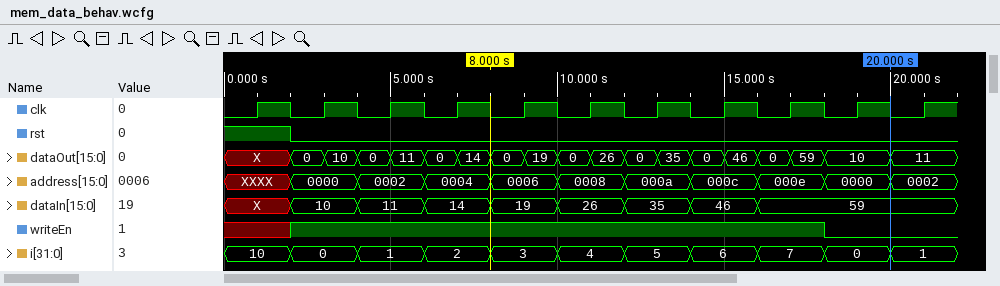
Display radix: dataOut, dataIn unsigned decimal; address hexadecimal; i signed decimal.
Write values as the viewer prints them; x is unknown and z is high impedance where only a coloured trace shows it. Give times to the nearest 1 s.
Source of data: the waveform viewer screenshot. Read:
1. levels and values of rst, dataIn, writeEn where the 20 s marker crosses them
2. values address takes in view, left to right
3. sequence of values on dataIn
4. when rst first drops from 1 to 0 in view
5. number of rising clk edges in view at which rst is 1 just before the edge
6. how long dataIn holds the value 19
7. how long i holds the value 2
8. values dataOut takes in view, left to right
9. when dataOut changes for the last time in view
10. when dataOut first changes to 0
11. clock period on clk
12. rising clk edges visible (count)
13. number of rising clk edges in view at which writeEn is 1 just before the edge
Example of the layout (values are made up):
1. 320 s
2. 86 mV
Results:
1. rst=0, dataIn=59, writeEn=0
2. XXXX, 0000, 0002, 0004, 0006, 0008, 000a, 000c, 000e, 0000, 0002
3. X, 10, 11, 14, 19, 26, 35, 46, 59
4. 2 s
5. 1
6. 2 s
7. 2 s
8. X, 0, 10, 0, 11, 0, 14, 0, 19, 0, 26, 0, 35, 0, 46, 0, 59, 10, 11
9. 20 s
10. 2 s
11. 2 s
12. 11
13. 8
